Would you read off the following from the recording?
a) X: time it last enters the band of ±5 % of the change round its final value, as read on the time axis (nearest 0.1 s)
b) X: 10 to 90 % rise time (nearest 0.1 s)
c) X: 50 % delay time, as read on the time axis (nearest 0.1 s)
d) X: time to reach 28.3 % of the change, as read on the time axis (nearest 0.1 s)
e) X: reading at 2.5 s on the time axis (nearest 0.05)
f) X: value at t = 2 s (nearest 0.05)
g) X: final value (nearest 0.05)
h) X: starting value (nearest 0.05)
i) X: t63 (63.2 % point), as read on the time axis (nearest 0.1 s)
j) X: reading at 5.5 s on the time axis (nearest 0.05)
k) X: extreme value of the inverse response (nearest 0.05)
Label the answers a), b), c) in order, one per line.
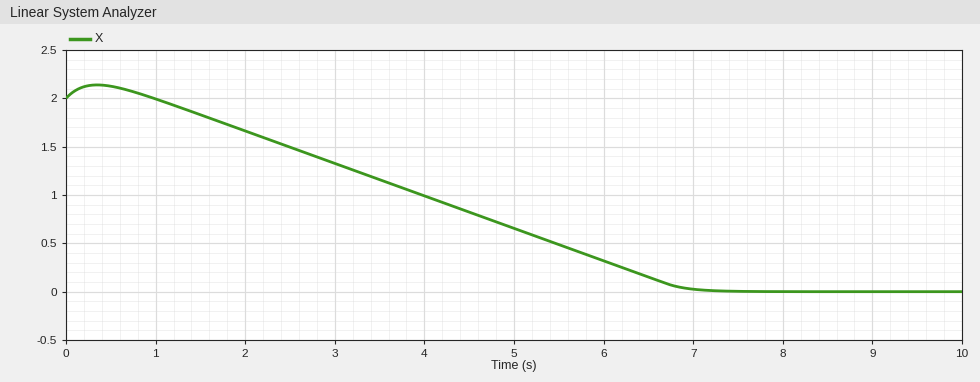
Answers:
a) 6.7 s
b) 4.8 s
c) 4.0 s
d) 2.7 s
e) 1.50
f) 1.65
g) 0.00
h) 2.00
i) 4.8 s
j) 0.50
k) 2.15
